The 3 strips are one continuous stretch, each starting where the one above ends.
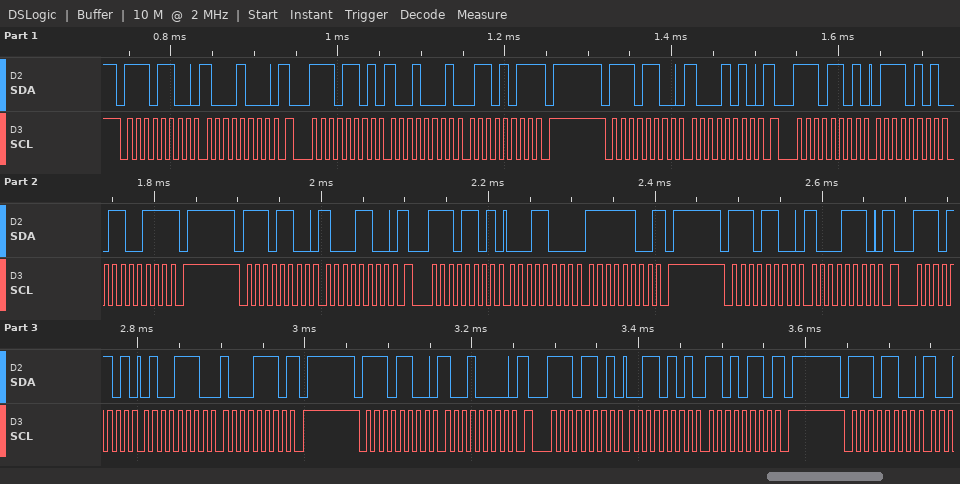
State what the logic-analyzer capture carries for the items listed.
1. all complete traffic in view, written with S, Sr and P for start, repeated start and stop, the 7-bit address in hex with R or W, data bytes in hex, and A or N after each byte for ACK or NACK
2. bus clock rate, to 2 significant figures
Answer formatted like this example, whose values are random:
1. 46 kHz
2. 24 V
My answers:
1. S 76W A 88 A Sr 76R A 91 A 6B N P S 76W A 8A A Sr 76R A 75 A 67 N P S 76W A 8C A Sr 76R A 18 A FC N P S 76W A 8E A Sr 76R A 4E A 8E N P S 76W A 90 A Sr 76R A 35 A D6 N P S 76W A
2. 100 kHz
